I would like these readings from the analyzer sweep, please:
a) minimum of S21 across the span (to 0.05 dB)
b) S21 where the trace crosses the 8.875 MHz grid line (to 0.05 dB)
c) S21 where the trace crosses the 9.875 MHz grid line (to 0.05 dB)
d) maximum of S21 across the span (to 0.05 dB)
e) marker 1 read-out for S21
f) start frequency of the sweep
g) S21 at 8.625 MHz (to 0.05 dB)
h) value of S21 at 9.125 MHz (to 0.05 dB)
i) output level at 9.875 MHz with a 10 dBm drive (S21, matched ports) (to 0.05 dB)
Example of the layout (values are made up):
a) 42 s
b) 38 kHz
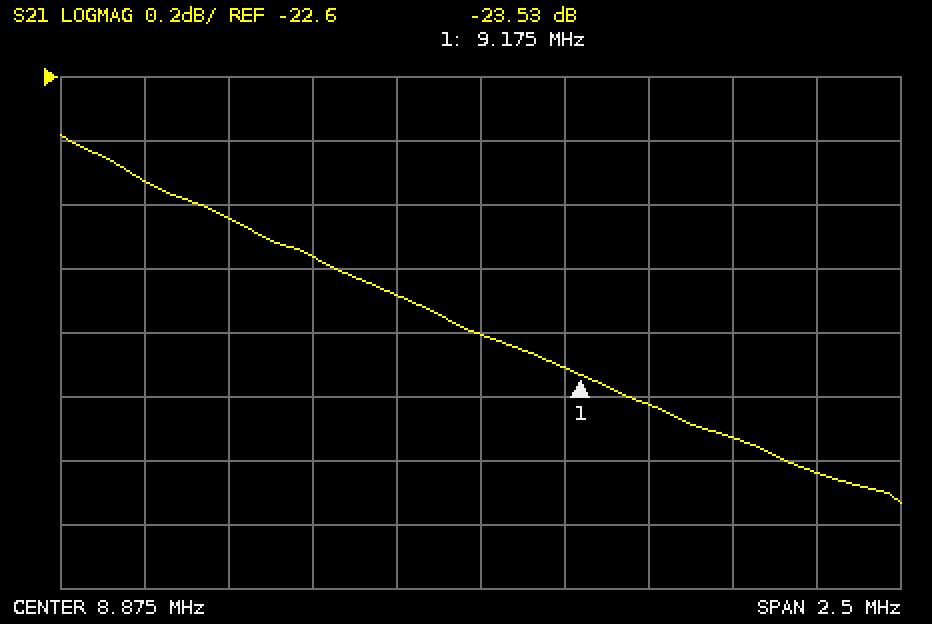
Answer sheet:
a) -23.95 dB
b) -23.40 dB
c) -23.85 dB
d) -22.80 dB
e) -23.53 dB
f) 7.625 MHz
g) -23.30 dB
h) -23.50 dB
i) -13.85 dBm
